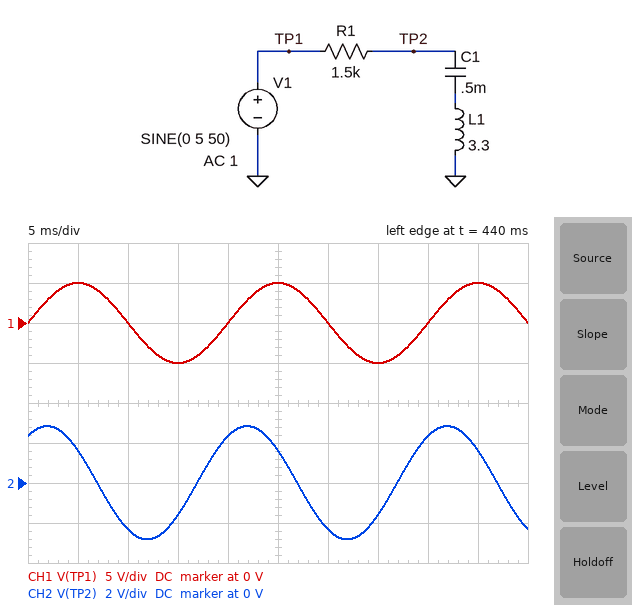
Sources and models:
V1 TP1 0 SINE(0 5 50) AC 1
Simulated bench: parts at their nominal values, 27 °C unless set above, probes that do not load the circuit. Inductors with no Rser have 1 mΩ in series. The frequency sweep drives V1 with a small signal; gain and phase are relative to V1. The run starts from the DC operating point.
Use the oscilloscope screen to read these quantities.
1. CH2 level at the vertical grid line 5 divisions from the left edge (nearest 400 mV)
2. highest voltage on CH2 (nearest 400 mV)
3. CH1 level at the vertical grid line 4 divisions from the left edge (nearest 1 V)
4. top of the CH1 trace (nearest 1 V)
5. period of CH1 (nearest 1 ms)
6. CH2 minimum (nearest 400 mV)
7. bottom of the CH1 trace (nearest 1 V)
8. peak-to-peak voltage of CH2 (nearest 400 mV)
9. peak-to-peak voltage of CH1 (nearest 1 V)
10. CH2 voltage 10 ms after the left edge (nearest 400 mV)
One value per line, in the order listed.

1.6 V
2.8 V
0 V
5 V
20 ms
-2.8 V
-5 V
5.6 V
10 V
-2.4 V
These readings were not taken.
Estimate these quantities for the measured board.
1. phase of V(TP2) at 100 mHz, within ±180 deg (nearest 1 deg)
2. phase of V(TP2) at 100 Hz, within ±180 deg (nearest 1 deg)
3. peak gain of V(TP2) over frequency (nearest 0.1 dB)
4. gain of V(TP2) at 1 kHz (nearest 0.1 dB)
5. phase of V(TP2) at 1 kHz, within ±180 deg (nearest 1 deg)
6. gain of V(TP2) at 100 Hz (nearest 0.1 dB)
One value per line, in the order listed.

-25 deg
36 deg
0 dB
0 dB
4 deg
-1.8 dB
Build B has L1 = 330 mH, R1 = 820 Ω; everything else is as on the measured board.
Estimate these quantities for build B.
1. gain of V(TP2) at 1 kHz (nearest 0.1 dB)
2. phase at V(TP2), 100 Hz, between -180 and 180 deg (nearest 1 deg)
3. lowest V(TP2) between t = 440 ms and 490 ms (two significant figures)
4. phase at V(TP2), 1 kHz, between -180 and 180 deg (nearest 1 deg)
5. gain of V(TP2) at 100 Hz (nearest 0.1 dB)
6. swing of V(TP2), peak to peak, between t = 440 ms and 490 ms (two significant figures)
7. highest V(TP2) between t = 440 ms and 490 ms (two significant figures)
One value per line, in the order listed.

-0.6 dB
76 deg
-580 mV
22 deg
-12.3 dB
1.2 V
600 mV
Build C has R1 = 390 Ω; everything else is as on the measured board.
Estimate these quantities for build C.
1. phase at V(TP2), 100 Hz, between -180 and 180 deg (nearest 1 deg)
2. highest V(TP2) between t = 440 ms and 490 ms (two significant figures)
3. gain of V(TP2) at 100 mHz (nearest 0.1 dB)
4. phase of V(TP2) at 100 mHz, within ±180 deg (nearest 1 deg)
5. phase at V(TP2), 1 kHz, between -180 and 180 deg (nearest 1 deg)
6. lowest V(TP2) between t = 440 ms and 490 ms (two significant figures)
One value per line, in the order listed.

11 deg
4.7 V
-0.1 dB
-7 deg
1 deg
-4.7 V
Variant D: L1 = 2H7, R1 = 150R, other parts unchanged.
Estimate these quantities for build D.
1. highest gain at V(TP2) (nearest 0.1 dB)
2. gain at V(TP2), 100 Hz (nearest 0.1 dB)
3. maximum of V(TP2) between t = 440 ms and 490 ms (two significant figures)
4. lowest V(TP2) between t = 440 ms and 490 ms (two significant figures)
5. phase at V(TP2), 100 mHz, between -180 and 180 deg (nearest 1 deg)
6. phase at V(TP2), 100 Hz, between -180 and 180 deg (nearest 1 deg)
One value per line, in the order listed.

0 dB
0 dB
4.9 V
-4.9 V
-3 deg
5 deg
